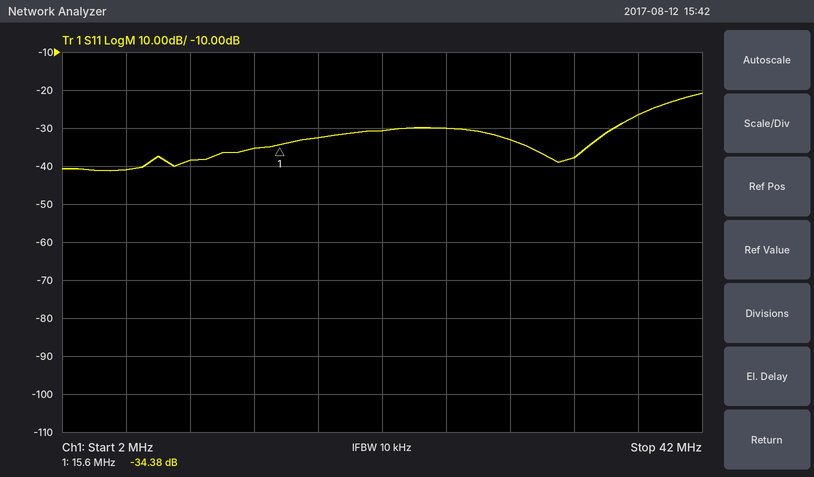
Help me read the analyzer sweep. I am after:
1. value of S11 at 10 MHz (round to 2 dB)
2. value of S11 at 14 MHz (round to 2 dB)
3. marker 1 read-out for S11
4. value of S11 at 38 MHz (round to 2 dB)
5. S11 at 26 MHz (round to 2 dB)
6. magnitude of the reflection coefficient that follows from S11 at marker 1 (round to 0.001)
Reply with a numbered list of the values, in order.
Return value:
1. -38 dB
2. -36 dB
3. -34.38 dB
4. -26 dB
5. -30 dB
6. 0.019
